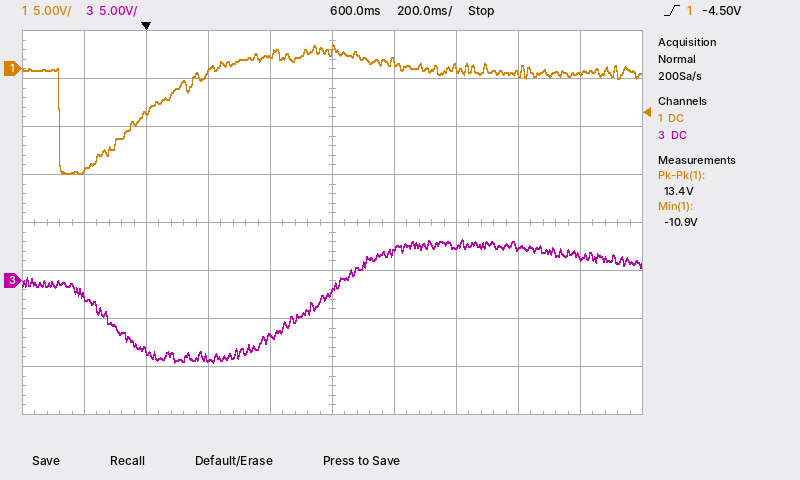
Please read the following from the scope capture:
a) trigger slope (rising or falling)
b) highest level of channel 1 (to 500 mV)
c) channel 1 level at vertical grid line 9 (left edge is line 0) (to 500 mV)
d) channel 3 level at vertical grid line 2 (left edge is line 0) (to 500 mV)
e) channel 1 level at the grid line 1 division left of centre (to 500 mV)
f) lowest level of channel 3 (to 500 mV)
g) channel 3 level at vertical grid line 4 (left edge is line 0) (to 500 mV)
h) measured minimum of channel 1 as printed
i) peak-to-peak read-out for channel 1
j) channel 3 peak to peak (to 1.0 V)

rising
2.5 V
-500 mV
-7.5 V
1.5 V
-8.5 V
-6.0 V
-10.9 V
13.4 V
13.0 V
